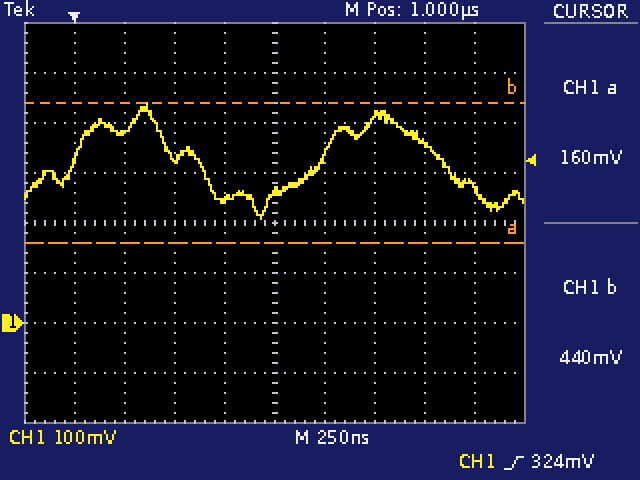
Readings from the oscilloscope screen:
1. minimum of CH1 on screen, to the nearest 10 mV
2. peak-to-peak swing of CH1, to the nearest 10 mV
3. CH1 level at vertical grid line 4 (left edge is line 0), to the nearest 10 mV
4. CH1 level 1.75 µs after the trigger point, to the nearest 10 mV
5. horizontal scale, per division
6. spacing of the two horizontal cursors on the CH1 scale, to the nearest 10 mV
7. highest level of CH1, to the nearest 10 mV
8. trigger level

210 mV
230 mV
250 mV
360 mV
250 ns
280 mV
440 mV
324 mV
